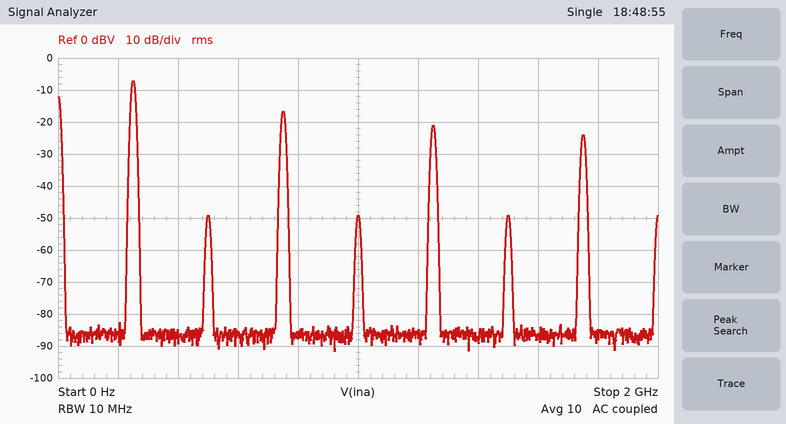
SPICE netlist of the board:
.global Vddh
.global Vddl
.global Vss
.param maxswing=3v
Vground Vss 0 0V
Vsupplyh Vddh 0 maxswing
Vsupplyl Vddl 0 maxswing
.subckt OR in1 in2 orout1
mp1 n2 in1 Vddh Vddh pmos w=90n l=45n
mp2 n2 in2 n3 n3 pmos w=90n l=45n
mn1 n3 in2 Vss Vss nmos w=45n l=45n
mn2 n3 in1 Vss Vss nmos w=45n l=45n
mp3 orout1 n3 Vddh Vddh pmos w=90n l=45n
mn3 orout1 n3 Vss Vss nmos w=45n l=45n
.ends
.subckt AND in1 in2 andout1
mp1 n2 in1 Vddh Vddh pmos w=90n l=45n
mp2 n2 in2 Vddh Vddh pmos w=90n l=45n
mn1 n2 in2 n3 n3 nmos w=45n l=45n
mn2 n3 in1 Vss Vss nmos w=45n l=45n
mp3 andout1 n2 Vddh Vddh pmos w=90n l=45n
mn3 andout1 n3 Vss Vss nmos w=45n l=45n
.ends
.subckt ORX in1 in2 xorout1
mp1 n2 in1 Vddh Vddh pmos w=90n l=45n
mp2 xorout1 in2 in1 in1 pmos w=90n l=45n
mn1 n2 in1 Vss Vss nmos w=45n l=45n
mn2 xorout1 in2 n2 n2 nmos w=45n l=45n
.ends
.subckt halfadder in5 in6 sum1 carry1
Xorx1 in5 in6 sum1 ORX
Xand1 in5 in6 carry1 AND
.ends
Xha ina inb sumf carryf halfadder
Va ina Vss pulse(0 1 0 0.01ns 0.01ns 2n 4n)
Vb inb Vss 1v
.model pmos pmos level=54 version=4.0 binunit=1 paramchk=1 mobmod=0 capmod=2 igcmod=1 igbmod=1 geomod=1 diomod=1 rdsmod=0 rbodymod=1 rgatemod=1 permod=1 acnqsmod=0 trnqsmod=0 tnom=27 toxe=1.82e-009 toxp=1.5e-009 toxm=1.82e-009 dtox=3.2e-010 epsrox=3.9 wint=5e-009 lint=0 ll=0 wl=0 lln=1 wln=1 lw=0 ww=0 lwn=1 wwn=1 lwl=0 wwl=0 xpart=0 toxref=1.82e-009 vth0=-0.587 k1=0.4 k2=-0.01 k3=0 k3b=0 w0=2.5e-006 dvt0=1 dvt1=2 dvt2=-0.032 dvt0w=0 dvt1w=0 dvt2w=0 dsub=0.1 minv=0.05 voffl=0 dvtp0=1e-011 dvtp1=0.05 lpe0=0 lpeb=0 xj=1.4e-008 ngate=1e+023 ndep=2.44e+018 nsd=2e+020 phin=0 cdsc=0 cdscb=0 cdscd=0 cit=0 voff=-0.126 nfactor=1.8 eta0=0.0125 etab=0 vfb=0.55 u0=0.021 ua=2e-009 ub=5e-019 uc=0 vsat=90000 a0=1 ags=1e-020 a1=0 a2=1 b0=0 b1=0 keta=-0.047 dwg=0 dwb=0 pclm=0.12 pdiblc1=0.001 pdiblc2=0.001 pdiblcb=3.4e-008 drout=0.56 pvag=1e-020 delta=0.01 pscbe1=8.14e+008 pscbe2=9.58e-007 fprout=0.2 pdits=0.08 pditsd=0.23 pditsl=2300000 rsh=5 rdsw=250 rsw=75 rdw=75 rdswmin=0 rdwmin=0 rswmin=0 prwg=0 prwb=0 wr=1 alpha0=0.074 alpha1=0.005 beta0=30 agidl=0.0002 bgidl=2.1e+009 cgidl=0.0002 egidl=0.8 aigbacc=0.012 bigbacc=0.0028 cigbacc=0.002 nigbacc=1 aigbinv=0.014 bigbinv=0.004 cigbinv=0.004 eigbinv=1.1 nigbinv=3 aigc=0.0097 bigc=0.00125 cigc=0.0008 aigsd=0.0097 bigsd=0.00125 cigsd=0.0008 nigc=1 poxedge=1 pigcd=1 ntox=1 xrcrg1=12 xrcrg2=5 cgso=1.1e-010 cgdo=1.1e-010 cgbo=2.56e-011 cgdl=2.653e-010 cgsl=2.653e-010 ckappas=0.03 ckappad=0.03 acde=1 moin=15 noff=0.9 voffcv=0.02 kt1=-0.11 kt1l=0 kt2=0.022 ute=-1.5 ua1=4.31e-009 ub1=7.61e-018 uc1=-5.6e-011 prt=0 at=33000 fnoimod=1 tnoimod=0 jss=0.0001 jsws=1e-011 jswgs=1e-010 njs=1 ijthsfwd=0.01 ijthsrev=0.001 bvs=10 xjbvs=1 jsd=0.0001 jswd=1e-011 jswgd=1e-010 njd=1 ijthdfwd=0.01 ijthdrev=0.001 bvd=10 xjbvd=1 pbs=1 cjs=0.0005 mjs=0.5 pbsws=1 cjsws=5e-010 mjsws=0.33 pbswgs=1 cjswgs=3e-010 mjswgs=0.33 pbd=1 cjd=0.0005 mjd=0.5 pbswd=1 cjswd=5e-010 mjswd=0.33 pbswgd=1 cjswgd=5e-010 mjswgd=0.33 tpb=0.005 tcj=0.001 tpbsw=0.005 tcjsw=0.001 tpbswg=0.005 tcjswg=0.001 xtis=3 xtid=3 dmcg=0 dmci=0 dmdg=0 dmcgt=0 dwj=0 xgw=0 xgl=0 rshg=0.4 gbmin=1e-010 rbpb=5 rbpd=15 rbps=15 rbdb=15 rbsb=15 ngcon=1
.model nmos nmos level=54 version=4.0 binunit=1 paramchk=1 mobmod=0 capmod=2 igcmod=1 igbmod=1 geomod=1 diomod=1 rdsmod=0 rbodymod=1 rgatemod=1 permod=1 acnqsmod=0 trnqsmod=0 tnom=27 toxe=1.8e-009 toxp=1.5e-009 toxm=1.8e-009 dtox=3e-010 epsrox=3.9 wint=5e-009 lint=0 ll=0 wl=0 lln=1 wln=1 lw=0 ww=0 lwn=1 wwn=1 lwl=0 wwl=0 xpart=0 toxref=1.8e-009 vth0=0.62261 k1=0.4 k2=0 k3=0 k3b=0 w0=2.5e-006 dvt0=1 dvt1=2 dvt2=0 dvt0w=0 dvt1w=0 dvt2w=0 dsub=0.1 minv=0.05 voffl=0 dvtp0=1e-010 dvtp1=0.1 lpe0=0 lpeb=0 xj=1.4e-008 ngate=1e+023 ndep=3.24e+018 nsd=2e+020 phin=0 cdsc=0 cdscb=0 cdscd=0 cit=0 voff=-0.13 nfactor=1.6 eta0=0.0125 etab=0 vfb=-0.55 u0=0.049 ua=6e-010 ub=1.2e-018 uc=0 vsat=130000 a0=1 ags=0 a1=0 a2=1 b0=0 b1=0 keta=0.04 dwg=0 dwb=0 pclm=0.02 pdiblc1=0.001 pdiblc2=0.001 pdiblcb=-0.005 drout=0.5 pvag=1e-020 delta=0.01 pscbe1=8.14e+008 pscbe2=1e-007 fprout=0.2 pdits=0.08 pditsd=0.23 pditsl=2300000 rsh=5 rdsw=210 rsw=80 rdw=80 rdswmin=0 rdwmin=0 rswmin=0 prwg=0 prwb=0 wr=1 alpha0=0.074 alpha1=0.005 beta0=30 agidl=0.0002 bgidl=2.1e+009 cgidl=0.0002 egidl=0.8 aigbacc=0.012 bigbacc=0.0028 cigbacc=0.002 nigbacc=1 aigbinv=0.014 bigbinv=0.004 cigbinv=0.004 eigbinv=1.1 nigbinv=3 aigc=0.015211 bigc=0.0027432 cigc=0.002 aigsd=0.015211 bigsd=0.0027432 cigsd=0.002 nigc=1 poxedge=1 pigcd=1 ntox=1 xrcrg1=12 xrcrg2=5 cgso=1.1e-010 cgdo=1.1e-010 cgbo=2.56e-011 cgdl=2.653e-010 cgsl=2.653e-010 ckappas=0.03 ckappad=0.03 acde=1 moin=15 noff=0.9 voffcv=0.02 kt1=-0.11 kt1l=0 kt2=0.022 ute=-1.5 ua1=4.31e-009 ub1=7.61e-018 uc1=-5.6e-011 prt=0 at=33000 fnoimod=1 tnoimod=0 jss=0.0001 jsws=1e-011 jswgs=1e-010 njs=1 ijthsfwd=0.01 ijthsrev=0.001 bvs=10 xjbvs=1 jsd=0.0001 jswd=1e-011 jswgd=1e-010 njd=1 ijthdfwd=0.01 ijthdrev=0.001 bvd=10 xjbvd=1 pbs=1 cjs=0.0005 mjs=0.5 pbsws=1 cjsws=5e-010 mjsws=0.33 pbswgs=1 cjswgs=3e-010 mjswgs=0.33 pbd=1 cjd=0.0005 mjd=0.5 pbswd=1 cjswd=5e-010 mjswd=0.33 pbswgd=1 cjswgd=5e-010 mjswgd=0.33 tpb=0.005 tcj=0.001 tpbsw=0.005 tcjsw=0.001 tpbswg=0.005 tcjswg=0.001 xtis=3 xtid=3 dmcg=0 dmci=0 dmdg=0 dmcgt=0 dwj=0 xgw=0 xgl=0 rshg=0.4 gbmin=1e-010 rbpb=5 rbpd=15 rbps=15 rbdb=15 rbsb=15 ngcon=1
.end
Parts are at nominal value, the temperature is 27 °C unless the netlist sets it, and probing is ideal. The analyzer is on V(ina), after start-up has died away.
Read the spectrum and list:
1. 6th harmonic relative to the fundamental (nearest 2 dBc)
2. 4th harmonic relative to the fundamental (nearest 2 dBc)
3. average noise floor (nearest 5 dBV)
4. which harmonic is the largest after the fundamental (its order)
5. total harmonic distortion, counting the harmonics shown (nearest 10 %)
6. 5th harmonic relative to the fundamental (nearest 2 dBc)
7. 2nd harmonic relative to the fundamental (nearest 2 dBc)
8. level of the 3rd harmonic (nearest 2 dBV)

-42 dBc
-42 dBc
-85 dBV
3
40 %
-14 dBc
-42 dBc
-16 dBV
